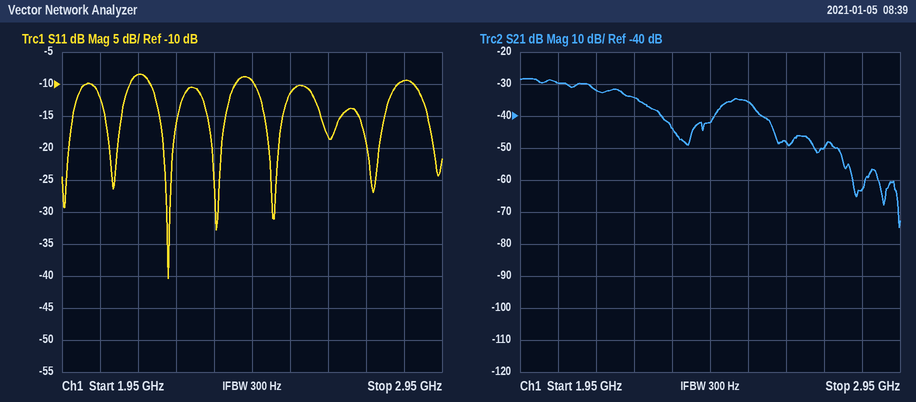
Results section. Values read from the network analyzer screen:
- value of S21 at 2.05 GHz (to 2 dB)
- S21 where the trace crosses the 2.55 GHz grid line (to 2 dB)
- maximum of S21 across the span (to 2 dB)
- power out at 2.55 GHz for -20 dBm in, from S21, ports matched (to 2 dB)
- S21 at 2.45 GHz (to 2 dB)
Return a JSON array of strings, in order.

["-30 dB", "-36 dB", "-28 dB", "-56 dBm", "-42 dB"]
